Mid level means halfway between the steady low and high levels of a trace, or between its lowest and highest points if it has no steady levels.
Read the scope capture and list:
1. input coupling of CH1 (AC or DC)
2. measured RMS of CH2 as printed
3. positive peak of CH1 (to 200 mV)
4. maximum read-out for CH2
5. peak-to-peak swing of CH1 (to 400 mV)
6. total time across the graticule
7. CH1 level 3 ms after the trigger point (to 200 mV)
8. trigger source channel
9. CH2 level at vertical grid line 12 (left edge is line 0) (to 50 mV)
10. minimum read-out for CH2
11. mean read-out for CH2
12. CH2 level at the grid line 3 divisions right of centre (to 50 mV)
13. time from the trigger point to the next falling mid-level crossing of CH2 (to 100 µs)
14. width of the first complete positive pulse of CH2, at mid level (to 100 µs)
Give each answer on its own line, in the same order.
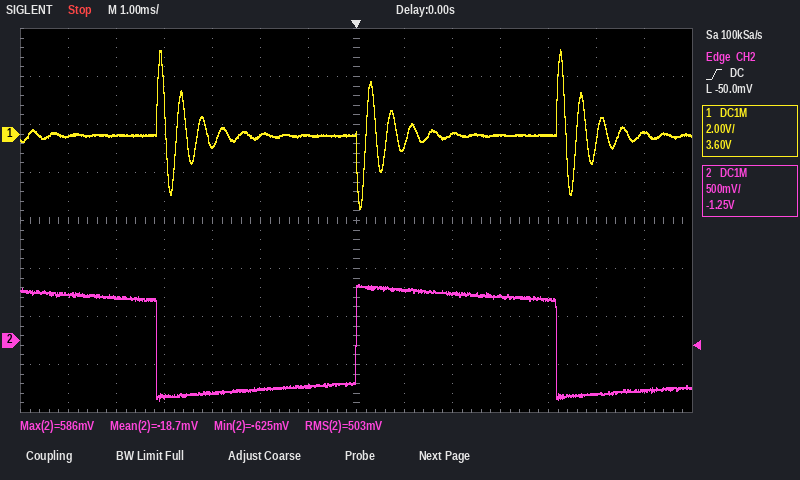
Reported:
DC
503 mV
3.6 V
586 mV
6.8 V
14 ms
0.0 V
CH2
-550 mV
-625 mV
-18.7 mV
450 mV
4.2 ms
4.2 ms
